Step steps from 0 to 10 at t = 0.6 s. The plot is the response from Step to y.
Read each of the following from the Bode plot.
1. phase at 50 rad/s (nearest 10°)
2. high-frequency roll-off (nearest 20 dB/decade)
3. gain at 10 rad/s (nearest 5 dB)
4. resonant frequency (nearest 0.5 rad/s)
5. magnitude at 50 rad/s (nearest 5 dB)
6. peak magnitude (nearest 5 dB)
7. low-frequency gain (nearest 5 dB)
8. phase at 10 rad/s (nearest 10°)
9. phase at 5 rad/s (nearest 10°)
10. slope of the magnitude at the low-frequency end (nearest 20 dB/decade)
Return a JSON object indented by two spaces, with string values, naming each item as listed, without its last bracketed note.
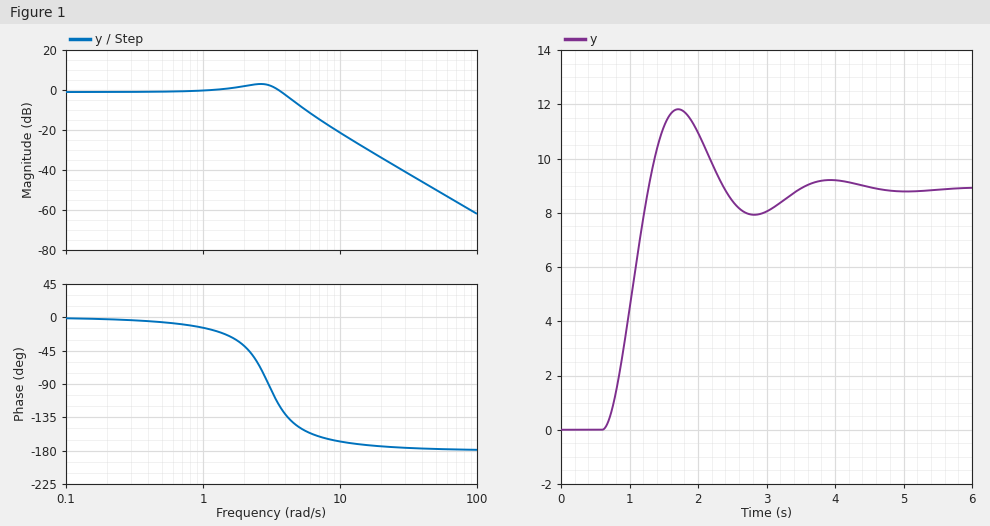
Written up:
{
  "phase at 50 rad/s": "-180°",
  "high-frequency roll-off": "-40 dB/decade",
  "gain at 10 rad/s": "-20 dB",
  "resonant frequency": "2.5 rad/s",
  "magnitude at 50 rad/s": "-50 dB",
  "peak magnitude": "5 dB",
  "low-frequency gain": "0 dB",
  "phase at 10 rad/s": "-170°",
  "phase at 5 rad/s": "-150°",
  "slope of the magnitude at the low-frequency end": "0 dB/decade"
}
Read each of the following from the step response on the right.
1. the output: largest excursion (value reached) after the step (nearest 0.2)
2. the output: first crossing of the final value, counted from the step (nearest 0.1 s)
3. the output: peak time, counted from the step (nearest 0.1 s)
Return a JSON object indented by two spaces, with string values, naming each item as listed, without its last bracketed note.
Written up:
{
  "the output: largest excursion (value reached) after the step": "11.8",
  "the output: first crossing of the final value, counted from the step": "0.7 s",
  "the output: peak time, counted from the step": "1.1 s"
}
